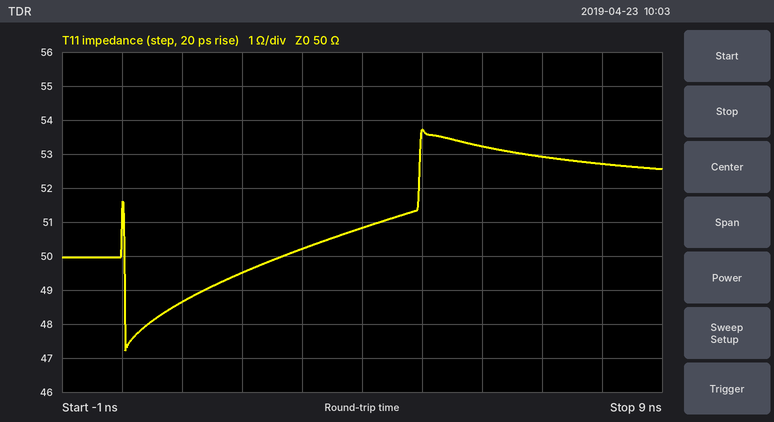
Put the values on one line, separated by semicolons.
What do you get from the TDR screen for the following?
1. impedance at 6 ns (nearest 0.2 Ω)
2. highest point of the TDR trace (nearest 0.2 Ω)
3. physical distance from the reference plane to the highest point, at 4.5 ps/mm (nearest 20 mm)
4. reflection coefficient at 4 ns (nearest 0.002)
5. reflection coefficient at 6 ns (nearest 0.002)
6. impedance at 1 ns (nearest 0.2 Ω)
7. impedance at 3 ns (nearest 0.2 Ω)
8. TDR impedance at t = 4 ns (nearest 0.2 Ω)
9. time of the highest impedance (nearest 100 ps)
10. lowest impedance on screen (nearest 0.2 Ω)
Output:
53.2 Ω; 53.8 Ω; 560 mm; +0.008; +0.032; 48.6 Ω; 50.2 Ω; 50.8 Ω; 5.0 ns; 47.2 Ω
